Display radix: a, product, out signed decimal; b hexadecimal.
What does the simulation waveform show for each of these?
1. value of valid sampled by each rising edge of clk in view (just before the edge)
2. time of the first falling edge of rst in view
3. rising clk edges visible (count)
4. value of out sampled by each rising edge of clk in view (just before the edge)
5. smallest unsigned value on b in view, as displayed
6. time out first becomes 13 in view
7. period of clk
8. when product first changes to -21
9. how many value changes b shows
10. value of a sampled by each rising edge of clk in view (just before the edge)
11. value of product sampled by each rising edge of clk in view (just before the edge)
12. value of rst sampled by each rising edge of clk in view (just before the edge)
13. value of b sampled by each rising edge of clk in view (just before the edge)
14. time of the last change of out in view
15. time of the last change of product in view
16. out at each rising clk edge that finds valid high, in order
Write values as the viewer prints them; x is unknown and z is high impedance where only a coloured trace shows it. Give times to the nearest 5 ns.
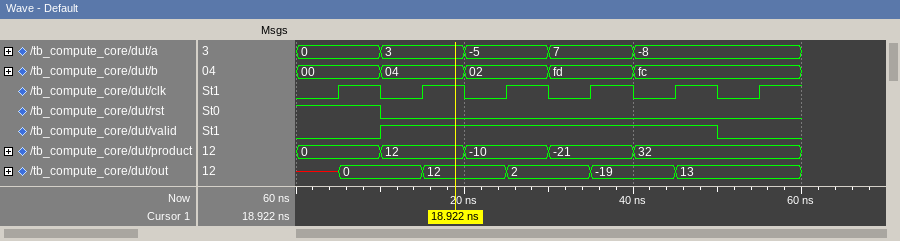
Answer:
0 1 1 1 1 0
10 ns
6
x, 0, 12, 2, -19, 13
00
45 ns
10 ns
30 ns
4
0, 3, -5, 7, -8, -8
0, 12, -10, -21, 32, 32
1 0 0 0 0 0
00, 04, 02, fd, fc, fc
45 ns
40 ns
0, 12, 2, -19
